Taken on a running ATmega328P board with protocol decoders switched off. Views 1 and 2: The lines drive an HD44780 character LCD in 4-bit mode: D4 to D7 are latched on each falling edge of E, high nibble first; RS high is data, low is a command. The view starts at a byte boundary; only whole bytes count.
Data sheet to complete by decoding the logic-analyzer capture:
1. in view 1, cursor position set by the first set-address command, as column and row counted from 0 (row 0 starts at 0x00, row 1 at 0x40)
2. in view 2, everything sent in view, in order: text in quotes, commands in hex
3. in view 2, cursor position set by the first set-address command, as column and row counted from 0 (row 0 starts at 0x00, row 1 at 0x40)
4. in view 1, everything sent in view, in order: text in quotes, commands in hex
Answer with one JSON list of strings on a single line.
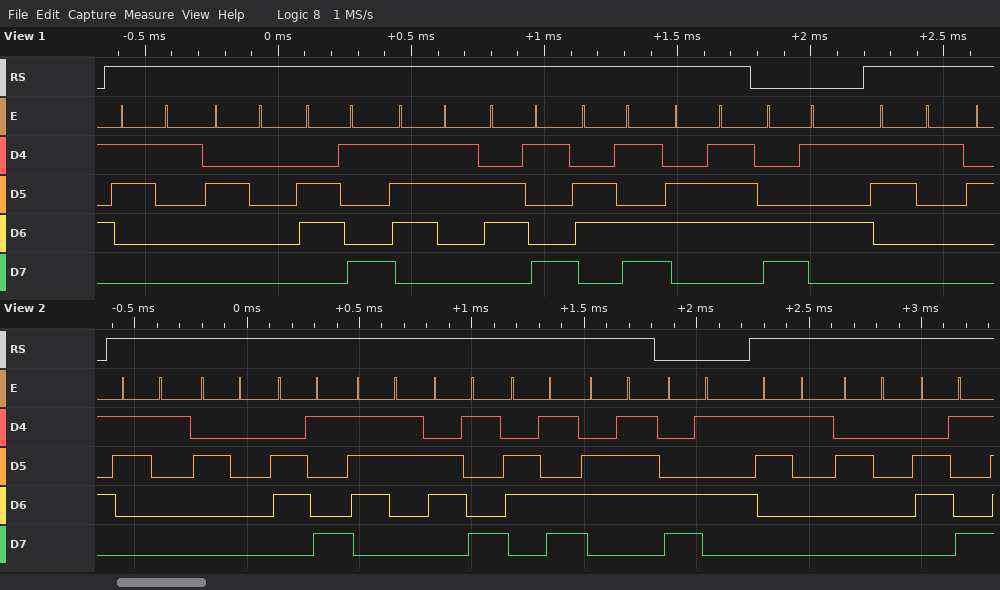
["column 5, row 1", "\"1 isimg\" 0xC5 \"1 i\"", "column 5, row 1", "\"1 isimg\" 0xC5 \"1\""]
